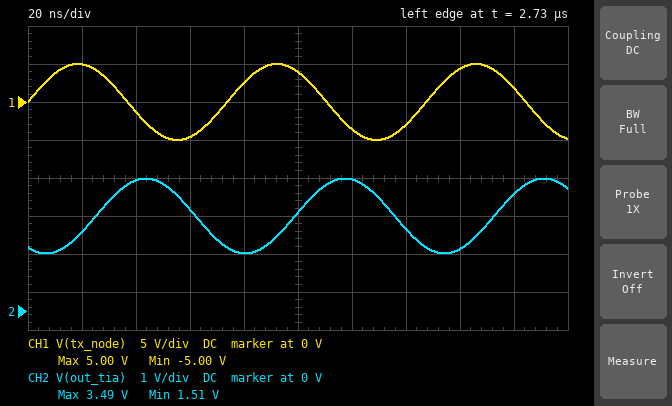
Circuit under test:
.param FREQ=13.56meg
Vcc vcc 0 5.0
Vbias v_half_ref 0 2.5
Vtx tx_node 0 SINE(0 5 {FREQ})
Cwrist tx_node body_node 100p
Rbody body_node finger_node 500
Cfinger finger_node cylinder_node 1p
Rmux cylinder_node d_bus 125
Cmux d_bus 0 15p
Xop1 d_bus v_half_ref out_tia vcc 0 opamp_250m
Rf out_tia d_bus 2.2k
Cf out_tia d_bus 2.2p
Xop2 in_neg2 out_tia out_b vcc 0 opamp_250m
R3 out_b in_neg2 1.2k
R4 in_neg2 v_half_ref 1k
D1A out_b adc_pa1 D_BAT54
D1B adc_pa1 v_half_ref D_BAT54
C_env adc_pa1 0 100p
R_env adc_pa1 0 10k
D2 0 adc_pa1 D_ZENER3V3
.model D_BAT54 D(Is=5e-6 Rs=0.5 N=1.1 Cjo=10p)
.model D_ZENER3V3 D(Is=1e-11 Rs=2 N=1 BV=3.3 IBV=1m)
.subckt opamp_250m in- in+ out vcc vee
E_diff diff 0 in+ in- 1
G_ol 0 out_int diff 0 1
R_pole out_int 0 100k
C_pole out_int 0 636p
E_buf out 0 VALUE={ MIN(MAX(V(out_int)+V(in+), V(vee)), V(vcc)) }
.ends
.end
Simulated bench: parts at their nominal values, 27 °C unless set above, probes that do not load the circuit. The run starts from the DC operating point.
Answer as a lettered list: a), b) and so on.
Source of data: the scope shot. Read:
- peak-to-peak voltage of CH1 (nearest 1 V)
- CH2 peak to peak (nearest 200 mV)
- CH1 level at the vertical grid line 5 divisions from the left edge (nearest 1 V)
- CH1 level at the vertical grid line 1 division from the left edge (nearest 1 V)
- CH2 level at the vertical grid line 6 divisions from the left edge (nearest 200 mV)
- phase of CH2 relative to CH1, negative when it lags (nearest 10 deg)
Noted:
a) 10 V
b) 2.0 V
c) 4 V
d) 5 V
e) 3.4 V
f) -120 deg
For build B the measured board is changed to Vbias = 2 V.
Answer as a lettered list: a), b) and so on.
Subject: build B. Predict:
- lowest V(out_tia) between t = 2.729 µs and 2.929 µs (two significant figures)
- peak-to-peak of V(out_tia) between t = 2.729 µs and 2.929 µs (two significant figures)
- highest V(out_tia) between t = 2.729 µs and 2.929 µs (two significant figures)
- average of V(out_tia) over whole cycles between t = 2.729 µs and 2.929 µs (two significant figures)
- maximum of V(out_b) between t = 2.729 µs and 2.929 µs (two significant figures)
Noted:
a) 1.0 V
b) 2.0 V
c) 3.0 V
d) 2.0 V
e) 4.2 V
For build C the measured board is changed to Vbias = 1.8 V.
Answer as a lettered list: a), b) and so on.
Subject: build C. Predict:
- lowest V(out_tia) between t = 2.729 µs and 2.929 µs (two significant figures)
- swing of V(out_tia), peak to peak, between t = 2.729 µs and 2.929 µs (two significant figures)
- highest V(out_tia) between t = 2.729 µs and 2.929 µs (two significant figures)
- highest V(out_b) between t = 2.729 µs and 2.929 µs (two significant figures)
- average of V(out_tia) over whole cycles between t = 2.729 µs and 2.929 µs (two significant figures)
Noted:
a) 810 mV
b) 2.0 V
c) 2.8 V
d) 4.0 V
e) 1.8 V
